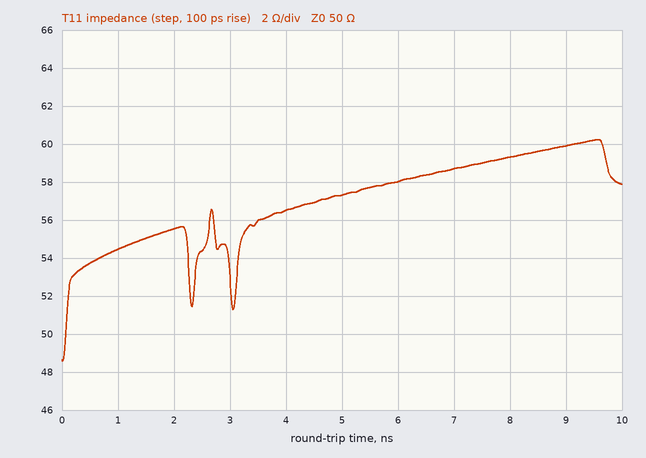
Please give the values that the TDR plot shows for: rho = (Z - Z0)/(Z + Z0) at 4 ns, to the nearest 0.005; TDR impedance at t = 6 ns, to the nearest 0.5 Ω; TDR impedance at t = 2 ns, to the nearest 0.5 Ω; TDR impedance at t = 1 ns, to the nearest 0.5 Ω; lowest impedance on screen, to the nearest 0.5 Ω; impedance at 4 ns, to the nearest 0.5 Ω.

+0.060
58.0 Ω
55.5 Ω
54.5 Ω
48.5 Ω
56.5 Ω
